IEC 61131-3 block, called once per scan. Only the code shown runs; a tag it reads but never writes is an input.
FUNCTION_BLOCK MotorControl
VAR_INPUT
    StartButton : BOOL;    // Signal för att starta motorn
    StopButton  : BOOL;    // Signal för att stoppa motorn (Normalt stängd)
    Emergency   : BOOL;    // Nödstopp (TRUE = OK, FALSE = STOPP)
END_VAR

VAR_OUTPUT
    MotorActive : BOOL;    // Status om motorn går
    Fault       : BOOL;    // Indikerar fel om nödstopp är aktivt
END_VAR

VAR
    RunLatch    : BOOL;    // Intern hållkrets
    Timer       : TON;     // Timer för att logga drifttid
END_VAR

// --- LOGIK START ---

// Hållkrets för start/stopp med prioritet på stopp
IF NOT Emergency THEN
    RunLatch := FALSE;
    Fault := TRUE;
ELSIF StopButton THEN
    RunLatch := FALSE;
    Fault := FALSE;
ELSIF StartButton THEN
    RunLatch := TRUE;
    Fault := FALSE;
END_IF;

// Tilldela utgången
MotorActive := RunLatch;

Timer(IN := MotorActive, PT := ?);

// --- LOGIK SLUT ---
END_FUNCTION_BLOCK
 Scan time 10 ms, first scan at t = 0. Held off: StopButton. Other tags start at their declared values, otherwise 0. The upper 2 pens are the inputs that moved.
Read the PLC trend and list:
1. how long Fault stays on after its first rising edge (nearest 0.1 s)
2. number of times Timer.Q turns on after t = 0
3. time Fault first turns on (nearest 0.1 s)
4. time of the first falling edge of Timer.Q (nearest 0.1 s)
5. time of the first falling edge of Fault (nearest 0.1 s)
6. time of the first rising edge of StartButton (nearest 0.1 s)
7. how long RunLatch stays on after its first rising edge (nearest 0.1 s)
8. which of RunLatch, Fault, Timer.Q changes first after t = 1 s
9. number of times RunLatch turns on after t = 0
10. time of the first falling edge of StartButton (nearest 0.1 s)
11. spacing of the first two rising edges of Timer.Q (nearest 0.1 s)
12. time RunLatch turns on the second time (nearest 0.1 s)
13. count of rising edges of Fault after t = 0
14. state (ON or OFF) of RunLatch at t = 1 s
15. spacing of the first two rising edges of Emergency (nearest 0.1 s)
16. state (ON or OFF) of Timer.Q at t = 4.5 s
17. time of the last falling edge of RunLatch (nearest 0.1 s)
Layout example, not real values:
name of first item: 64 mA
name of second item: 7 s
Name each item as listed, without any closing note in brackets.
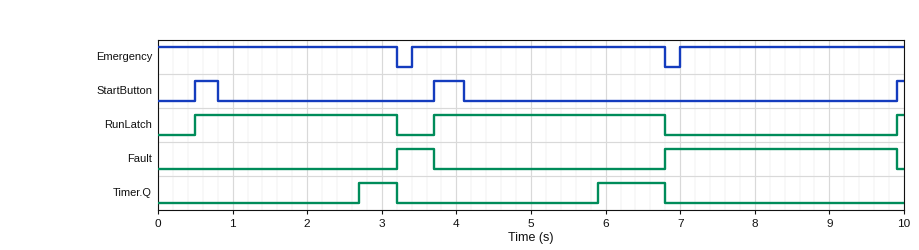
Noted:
how long Fault stays on after its first rising edge: 0.5 s
number of times Timer.Q turns on after t = 0: 2
time Fault first turns on: 3.2 s
time of the first falling edge of Timer.Q: 3.2 s
time of the first falling edge of Fault: 3.7 s
time of the first rising edge of StartButton: 0.5 s
how long RunLatch stays on after its first rising edge: 2.7 s
which of RunLatch, Fault, Timer.Q changes first after t = 1 s: Timer.Q
number of times RunLatch turns on after t = 0: 3
time of the first falling edge of StartButton: 0.8 s
spacing of the first two rising edges of Timer.Q: 3.2 s
time RunLatch turns on the second time: 3.7 s
count of rising edges of Fault after t = 0: 2
state (ON or OFF) of RunLatch at t = 1 s: ON
spacing of the first two rising edges of Emergency: 3.6 s
state (ON or OFF) of Timer.Q at t = 4.5 s: OFF
time of the last falling edge of RunLatch: 6.8 s
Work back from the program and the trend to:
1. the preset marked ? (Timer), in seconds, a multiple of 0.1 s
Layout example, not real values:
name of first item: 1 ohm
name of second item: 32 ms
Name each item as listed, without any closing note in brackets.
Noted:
the preset marked ? (Timer), in seconds, a multiple of 0.1 s: 2.2 s
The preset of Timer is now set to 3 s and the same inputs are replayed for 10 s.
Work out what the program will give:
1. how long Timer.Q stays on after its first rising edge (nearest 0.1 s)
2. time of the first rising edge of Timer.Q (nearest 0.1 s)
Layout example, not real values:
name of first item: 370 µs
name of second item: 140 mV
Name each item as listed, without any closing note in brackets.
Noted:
how long Timer.Q stays on after its first rising edge: 0.1 s
time of the first rising edge of Timer.Q: 6.7 s
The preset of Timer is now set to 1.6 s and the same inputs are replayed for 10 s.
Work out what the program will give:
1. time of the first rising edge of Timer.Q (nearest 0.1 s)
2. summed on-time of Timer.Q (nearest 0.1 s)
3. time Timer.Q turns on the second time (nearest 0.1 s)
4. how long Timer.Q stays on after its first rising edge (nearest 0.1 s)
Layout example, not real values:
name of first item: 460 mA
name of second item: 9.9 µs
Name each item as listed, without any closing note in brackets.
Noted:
time of the first rising edge of Timer.Q: 2.1 s
summed on-time of Timer.Q: 2.6 s
time Timer.Q turns on the second time: 5.3 s
how long Timer.Q stays on after its first rising edge: 1.1 s
